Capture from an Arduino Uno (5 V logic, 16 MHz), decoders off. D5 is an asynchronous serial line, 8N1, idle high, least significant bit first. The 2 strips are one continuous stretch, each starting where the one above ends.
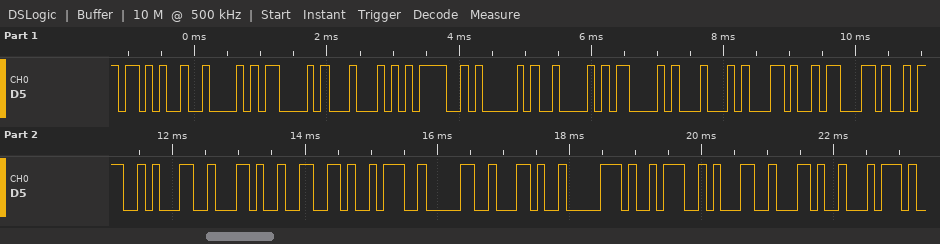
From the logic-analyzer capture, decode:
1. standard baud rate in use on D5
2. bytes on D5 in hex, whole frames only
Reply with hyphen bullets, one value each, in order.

- 9600 baud
- 2B 42 43 44 3D 41 42 43 44 2C 63 3A 31 2C 66 3A 30 2C 70 3A 31 2C 74
